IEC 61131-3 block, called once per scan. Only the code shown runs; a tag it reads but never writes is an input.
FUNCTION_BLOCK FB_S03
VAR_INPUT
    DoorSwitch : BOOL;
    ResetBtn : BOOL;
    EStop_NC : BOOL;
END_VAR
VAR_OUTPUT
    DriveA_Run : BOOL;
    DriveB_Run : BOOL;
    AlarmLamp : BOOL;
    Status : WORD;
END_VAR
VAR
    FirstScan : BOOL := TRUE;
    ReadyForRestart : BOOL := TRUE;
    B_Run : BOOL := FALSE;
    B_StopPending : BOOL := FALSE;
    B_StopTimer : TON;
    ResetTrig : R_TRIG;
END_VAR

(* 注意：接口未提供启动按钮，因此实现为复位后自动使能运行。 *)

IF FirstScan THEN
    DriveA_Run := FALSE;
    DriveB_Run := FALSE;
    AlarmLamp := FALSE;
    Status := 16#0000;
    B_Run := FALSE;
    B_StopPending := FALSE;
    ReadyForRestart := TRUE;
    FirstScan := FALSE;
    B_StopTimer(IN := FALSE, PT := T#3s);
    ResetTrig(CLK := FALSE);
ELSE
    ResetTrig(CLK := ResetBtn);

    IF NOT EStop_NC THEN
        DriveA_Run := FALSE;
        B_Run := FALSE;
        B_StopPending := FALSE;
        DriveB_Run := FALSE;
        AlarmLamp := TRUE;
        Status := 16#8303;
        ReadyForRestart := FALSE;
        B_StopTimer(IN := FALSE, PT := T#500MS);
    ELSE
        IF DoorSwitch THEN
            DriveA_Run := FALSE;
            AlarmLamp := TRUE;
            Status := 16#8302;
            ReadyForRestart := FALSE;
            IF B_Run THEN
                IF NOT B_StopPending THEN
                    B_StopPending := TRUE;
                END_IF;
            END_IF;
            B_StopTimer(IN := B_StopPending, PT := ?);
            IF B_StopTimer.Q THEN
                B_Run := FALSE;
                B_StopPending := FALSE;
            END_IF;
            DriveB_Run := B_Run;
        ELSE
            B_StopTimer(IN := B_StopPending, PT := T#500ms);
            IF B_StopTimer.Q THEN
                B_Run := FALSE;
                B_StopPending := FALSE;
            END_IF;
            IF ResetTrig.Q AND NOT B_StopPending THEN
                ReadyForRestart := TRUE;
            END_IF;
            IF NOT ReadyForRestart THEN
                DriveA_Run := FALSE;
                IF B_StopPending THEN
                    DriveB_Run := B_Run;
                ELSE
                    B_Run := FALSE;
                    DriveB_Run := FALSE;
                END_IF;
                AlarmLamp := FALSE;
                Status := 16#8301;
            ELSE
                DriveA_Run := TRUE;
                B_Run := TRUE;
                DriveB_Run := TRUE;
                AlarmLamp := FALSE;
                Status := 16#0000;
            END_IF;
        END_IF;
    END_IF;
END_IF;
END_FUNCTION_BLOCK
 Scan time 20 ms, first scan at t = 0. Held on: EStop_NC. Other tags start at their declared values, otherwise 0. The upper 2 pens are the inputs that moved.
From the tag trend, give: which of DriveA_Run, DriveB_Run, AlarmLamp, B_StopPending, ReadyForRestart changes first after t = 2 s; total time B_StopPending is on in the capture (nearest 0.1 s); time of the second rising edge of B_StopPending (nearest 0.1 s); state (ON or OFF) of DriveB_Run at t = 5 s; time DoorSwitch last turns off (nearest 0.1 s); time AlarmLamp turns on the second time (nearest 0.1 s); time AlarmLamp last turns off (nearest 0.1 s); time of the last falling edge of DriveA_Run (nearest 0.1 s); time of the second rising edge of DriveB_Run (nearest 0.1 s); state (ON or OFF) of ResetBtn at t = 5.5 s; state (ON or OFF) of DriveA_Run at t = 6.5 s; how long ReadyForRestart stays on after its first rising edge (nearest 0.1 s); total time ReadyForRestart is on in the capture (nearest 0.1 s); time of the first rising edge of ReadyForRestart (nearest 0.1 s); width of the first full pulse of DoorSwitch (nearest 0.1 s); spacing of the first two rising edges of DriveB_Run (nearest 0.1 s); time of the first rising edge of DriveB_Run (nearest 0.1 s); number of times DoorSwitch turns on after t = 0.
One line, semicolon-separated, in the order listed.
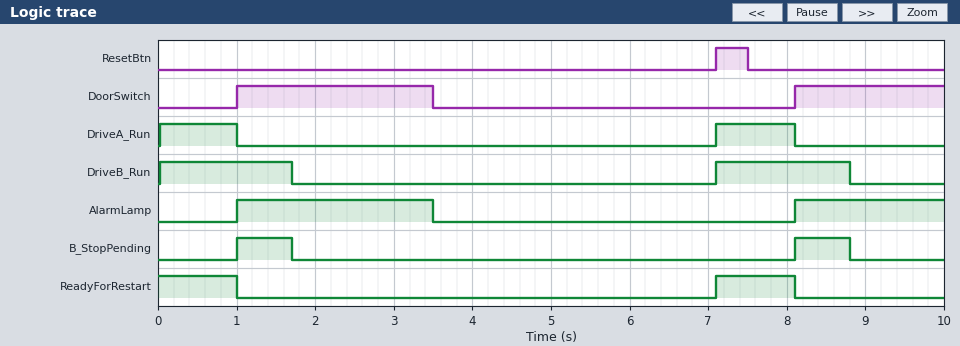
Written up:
AlarmLamp; 1.4 s; 8.1 s; OFF; 3.5 s; 8.1 s; 3.5 s; 8.1 s; 7.1 s; OFF; OFF; 1.0 s; 2.0 s; 7.1 s; 2.5 s; 7.1 s; 0.0 s; 2
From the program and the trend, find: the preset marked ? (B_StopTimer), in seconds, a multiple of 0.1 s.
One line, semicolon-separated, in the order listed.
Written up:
0.7 s
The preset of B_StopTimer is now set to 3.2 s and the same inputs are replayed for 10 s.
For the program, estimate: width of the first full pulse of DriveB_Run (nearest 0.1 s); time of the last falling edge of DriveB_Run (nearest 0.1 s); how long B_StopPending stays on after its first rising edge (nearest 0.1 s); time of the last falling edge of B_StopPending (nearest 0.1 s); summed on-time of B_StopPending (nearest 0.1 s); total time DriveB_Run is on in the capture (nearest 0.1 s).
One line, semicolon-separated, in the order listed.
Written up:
3.5 s; 3.5 s; 2.5 s; 3.5 s; 4.4 s; 6.4 s
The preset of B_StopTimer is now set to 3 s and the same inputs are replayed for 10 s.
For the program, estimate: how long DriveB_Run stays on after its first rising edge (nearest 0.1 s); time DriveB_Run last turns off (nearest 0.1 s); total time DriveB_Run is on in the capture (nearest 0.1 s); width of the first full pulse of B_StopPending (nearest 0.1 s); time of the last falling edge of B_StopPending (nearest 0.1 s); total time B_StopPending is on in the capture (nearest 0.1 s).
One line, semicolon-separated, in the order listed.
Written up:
3.5 s; 3.5 s; 6.4 s; 2.5 s; 3.5 s; 4.4 s
